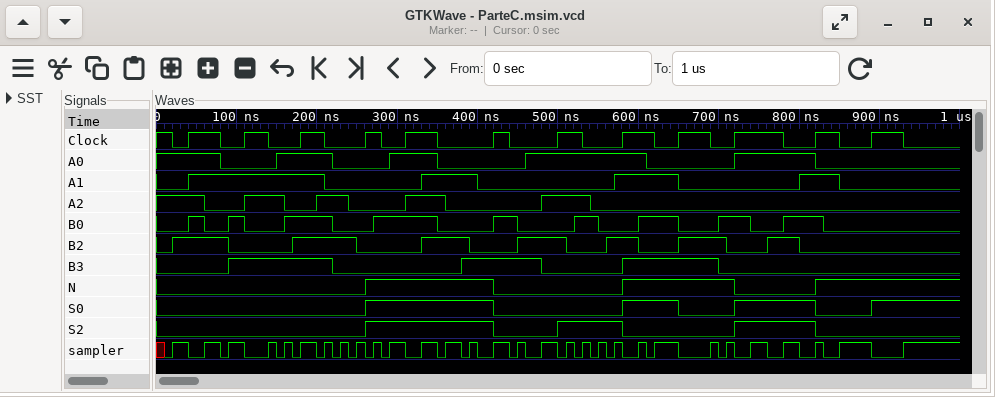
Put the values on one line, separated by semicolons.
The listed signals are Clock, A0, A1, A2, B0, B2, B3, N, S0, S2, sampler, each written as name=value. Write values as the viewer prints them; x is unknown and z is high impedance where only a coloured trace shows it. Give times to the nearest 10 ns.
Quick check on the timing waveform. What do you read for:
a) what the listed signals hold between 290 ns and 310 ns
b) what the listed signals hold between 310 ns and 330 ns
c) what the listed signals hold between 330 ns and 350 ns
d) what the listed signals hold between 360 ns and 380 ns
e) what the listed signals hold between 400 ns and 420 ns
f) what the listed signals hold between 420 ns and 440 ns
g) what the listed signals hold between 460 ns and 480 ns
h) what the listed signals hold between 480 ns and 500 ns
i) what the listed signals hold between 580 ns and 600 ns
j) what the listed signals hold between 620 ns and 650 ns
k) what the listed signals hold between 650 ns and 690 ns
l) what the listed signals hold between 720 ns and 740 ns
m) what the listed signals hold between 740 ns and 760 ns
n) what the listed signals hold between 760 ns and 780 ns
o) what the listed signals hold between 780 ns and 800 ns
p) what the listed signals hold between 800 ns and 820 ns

Clock=0, A0=1, A1=0, A2=0, B0=1, B2=0, B3=0, N=1, S0=1, S2=1, sampler=1; Clock=1, A0=1, A1=0, A2=1, B0=1, B2=0, B3=0, N=1, S0=1, S2=1, sampler=0; Clock=1, A0=1, A1=1, A2=1, B0=1, B2=1, B3=0, N=1, S0=1, S2=1, sampler=1; Clock=0, A0=0, A1=1, A2=0, B0=0, B2=1, B3=0, N=1, S0=1, S2=1, sampler=1; Clock=0, A0=0, A1=0, A2=0, B0=0, B2=0, B3=1, N=1, S0=1, S2=1, sampler=0; Clock=1, A0=0, A1=0, A2=0, B0=1, B2=0, B3=1, N=0, S0=0, S2=0, sampler=1; Clock=0, A0=1, A1=0, A2=0, B0=0, B2=1, B3=1, N=0, S0=0, S2=0, sampler=0; Clock=0, A0=1, A1=0, A2=1, B0=0, B2=1, B3=0, N=0, S0=0, S2=0, sampler=1; Clock=1, A0=1, A1=1, A2=0, B0=0, B2=1, B3=1, N=1, S0=1, S2=0, sampler=0; Clock=0, A0=0, A1=1, A2=0, B0=1, B2=0, B3=1, N=1, S0=1, S2=0, sampler=1; Clock=1, A0=0, A1=0, A2=0, B0=0, B2=1, B3=1, N=1, S0=0, S2=0, sampler=0; Clock=1, A0=1, A1=0, A2=0, B0=1, B2=0, B3=0, N=0, S0=1, S2=1, sampler=0; Clock=1, A0=1, A1=0, A2=0, B0=0, B2=0, B3=0, N=0, S0=1, S2=1, sampler=1; Clock=1, A0=1, A1=0, A2=0, B0=0, B2=1, B3=0, N=0, S0=1, S2=1, sampler=0; Clock=0, A0=1, A1=0, A2=0, B0=1, B2=1, B3=0, N=0, S0=1, S2=1, sampler=1; Clock=0, A0=1, A1=1, A2=0, B0=1, B2=0, B3=0, N=0, S0=1, S2=1, sampler=0
